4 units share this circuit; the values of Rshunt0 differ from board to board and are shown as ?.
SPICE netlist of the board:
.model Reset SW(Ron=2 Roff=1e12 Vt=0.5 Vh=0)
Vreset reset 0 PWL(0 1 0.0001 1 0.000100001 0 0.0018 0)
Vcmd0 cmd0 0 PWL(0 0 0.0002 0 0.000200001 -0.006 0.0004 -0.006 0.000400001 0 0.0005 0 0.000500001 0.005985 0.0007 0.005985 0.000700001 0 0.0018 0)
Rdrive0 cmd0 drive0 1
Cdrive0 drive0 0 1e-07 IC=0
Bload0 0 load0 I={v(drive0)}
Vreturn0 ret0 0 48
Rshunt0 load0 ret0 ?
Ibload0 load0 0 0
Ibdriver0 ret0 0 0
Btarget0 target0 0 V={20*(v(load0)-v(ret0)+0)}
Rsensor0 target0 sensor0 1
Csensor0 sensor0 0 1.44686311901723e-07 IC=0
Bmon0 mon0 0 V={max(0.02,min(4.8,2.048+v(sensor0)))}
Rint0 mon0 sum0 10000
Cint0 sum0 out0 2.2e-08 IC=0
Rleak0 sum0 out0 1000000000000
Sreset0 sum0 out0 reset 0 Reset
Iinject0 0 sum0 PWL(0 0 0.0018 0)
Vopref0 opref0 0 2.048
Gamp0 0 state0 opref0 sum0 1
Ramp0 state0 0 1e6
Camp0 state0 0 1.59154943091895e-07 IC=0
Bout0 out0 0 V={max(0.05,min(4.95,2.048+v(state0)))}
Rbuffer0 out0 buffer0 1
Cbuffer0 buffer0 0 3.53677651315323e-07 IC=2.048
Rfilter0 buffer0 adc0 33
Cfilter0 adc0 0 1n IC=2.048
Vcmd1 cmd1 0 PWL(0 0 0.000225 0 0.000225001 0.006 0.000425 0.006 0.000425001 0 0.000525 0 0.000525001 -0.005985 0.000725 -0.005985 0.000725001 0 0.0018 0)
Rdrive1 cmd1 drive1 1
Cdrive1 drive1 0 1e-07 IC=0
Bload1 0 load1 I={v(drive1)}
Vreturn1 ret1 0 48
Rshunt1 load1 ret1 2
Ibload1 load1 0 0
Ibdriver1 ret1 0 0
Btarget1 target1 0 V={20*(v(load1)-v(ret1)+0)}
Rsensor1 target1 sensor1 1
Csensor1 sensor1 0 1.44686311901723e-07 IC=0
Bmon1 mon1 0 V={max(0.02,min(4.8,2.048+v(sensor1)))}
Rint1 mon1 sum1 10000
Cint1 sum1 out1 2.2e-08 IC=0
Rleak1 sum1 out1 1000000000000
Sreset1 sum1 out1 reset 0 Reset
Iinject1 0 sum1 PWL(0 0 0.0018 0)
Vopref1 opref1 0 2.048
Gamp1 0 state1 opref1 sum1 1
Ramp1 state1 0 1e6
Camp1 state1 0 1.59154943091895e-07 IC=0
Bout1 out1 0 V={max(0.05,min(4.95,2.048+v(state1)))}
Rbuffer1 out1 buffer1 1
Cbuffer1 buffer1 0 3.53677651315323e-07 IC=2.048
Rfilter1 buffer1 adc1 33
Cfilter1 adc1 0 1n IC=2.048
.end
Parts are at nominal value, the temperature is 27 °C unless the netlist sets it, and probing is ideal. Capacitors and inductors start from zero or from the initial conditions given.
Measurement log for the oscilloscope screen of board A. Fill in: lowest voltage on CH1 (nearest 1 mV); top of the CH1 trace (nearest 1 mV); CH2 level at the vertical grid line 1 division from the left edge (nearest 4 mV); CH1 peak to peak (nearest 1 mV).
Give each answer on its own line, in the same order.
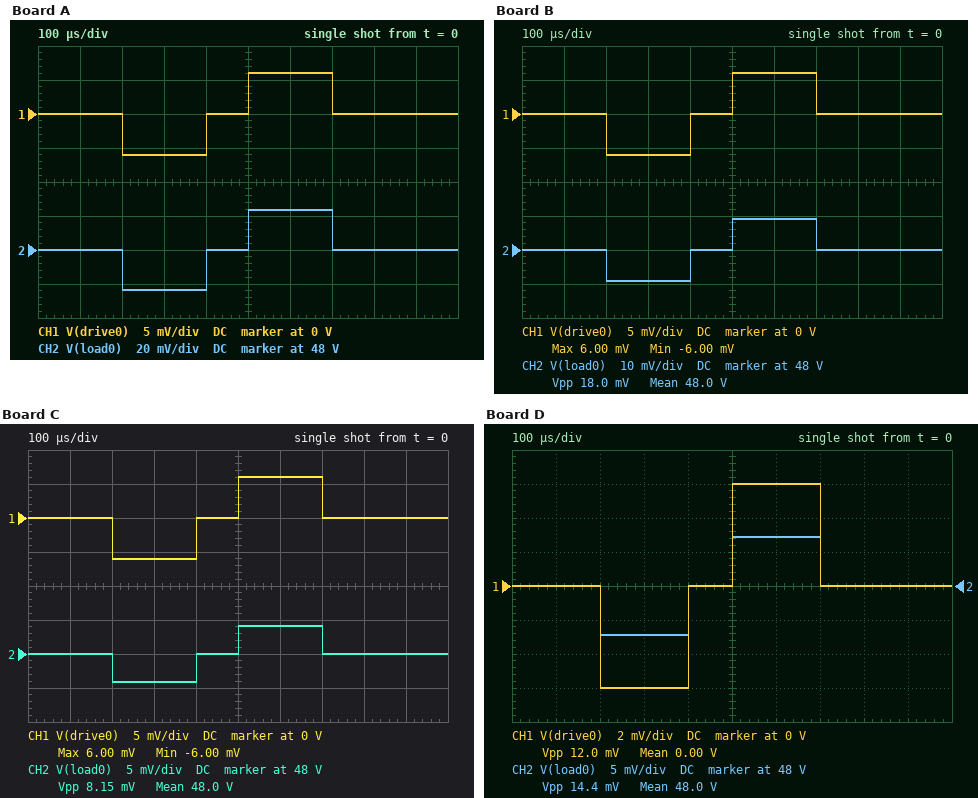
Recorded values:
-6 mV
6 mV
48.000 V
12 mV
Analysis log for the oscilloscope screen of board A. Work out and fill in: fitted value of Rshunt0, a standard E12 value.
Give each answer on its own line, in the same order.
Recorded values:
3.9 Ω
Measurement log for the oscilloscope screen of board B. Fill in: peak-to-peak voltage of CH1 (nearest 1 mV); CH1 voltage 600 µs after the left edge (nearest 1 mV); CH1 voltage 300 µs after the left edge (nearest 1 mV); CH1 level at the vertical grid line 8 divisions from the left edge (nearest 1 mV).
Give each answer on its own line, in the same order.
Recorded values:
12 mV
6 mV
-6 mV
0 V
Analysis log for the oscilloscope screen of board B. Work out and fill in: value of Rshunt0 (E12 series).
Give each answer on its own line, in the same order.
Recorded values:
1.5 Ω
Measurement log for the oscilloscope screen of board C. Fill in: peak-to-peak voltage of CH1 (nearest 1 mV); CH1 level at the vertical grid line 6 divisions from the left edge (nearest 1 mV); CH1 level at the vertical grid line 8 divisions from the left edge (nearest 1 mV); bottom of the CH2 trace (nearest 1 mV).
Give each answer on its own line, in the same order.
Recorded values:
12 mV
6 mV
0 V
47.996 V
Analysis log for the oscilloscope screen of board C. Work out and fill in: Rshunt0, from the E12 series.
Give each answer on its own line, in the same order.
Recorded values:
0.68 Ω
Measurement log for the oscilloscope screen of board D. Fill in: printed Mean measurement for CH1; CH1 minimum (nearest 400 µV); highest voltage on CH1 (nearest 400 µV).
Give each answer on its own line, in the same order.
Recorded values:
0.00 V
-6.0 mV
6.0 mV
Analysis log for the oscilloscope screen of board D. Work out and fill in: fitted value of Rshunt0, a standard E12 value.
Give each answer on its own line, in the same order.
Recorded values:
1.2 Ω
